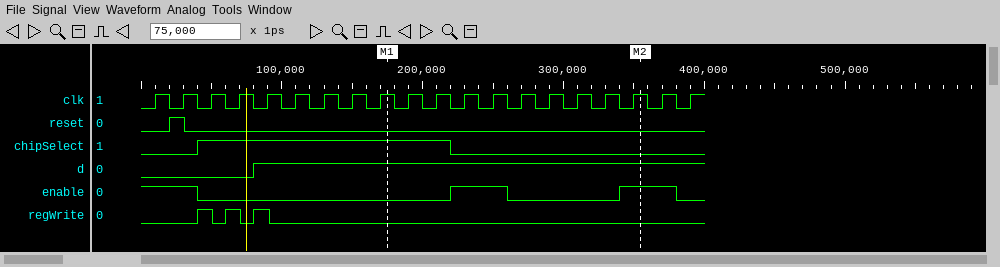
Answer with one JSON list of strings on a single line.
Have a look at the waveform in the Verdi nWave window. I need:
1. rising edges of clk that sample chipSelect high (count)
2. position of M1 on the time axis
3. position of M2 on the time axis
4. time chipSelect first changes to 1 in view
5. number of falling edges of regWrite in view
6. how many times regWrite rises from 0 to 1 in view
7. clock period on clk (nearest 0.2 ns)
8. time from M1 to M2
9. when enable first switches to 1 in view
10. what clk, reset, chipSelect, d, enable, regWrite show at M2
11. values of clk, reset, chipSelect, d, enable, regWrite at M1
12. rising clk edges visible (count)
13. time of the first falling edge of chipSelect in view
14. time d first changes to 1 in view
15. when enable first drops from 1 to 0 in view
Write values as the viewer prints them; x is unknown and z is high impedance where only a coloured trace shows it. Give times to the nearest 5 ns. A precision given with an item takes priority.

["9", "175 ns", "355 ns", "40 ns", "3", "3", "20 ns", "180 ns", "220 ns", "clk=1, reset=0, chipSelect=0, d=1, enable=1, regWrite=0", "clk=1, reset=0, chipSelect=1, d=1, enable=0, regWrite=0", "20", "220 ns", "80 ns", "40 ns"]
